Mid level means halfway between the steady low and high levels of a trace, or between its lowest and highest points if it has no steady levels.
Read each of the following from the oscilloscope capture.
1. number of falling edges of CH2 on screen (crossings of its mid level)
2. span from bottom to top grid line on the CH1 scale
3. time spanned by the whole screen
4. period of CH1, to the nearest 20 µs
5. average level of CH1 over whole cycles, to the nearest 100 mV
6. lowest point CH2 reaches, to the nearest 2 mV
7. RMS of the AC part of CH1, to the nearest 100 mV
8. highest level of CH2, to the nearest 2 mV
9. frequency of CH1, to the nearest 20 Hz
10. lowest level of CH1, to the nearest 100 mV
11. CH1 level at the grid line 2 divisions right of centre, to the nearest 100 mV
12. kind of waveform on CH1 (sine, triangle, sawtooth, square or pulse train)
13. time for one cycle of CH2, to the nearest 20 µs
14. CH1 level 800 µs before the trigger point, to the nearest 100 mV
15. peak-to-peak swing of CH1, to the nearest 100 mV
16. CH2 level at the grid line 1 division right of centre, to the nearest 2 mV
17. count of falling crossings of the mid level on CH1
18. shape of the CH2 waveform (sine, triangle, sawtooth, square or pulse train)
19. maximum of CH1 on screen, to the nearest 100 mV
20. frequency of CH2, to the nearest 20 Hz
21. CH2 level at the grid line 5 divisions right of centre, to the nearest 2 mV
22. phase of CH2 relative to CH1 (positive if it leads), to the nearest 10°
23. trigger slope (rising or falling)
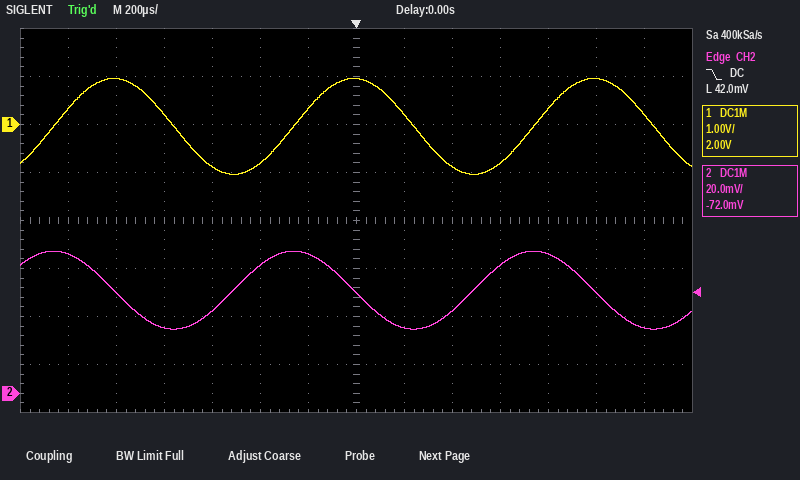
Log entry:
3
8 V
2.8 ms
1.00 ms
0.0 V
26 mV
700 mV
60 mV
1.00 kHz
-1.0 V
-900 mV
sine
1.00 ms
200 mV
2.0 V
28 mV
3
sine
1.0 V
1.00 kHz
42 mV
+90°
falling
